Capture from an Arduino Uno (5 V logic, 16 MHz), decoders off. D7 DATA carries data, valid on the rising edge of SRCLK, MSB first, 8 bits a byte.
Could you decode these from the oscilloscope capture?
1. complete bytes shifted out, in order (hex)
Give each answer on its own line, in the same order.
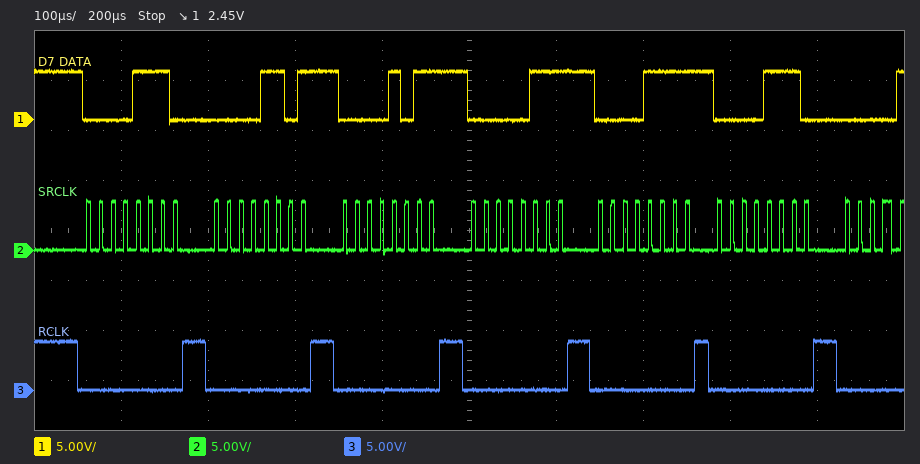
0E 0D 0B 07 0F 0E
